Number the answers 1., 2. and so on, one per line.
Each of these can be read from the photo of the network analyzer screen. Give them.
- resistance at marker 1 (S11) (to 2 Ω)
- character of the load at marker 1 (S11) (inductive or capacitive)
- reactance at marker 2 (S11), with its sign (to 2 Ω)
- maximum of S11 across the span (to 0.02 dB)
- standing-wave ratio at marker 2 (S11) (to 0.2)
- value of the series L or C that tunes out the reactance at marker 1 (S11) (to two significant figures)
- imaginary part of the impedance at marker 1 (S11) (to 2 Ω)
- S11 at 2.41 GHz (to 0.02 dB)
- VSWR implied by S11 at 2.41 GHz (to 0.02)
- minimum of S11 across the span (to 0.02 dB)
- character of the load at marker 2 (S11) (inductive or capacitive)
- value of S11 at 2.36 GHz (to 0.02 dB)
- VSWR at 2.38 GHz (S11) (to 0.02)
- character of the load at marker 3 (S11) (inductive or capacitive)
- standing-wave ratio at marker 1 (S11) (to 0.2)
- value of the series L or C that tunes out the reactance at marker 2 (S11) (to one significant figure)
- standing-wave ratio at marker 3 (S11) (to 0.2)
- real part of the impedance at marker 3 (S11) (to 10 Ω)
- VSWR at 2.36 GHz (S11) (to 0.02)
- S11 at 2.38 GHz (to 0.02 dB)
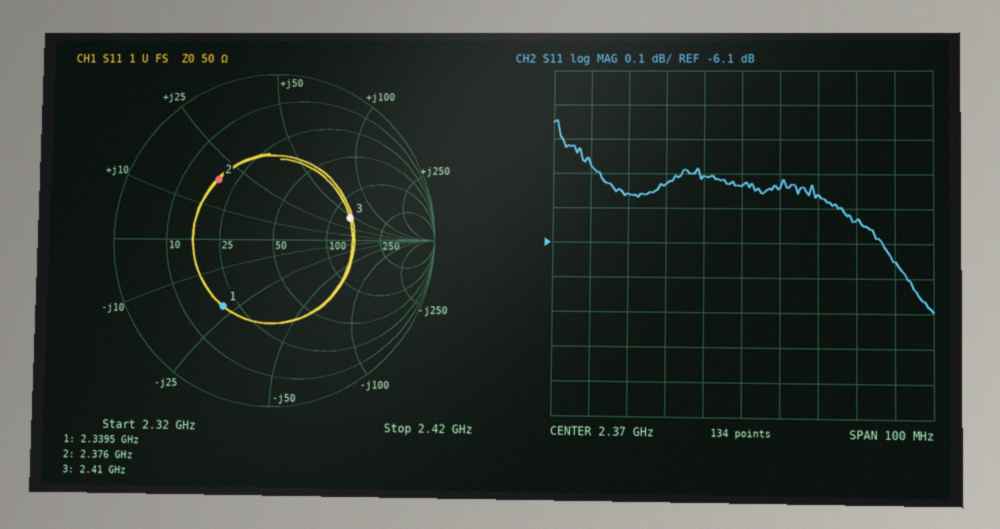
1. 20 Ω
2. capacitive
3. +18 Ω
4. -5.74 dB
5. 3.0
6. 1.5 nH
7. -22 Ω
8. -6.16 dB
9. 2.94
10. -6.30 dB
11. inductive
12. -5.90 dB
13. 3.04
14. inductive
15. 3.0
16. 4 pF
17. 3.0
18. 130 Ω
19. 3.06
20. -5.94 dB
